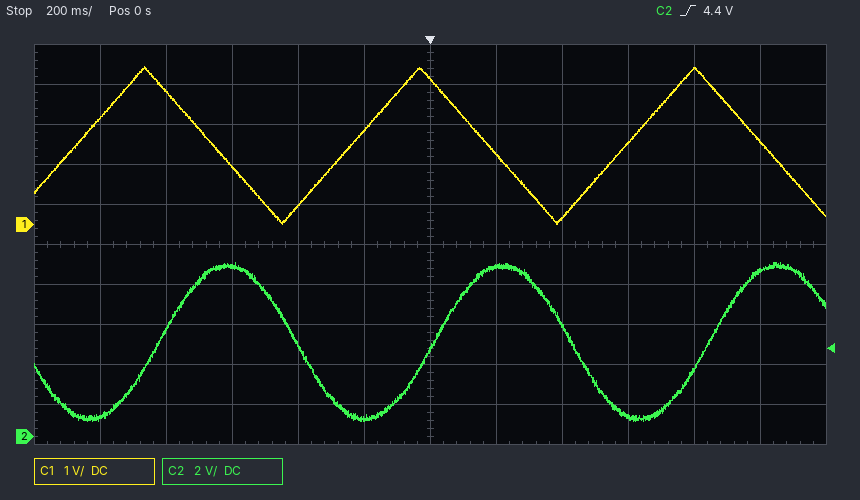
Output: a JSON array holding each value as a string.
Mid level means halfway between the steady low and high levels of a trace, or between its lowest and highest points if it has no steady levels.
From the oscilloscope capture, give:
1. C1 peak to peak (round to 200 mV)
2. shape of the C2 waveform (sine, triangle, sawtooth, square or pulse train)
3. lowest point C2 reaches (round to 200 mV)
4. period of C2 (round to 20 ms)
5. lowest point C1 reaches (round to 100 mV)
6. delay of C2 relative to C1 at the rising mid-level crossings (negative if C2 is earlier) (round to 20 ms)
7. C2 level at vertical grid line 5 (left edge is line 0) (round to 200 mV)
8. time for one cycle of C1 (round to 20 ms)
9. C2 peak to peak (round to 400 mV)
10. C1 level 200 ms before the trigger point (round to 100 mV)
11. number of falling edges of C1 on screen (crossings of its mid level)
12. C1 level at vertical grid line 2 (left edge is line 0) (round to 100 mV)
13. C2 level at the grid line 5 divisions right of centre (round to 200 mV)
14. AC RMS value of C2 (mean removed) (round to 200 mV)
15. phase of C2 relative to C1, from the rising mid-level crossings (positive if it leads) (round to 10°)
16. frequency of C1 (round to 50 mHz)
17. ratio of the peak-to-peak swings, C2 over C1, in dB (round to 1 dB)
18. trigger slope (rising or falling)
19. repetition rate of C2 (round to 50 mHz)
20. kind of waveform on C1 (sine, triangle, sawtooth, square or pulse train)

["4.0 V", "sine", "800 mV", "840 ms", "0.0 V", "+260 ms", "1.0 V", "840 ms", "8.0 V", "2.3 V", "3", "3.3 V", "8.2 V", "2.8 V", "-110°", "1.20 Hz", "6 dB", "rising", "1.20 Hz", "triangle"]
